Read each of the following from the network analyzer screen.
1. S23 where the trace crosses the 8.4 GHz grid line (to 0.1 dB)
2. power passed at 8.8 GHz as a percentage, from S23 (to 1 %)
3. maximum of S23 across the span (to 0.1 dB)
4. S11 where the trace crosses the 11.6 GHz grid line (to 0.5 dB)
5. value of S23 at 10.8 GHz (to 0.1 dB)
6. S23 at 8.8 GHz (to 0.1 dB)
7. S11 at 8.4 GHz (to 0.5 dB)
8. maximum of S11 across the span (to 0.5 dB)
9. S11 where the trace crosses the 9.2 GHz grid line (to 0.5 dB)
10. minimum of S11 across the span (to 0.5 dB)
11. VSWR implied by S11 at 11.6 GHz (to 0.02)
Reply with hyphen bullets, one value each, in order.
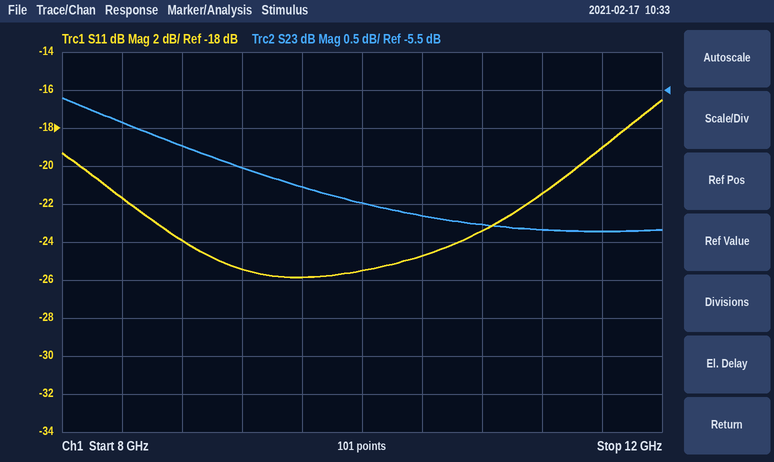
- -5.9 dB
- 24 %
- -5.6 dB
- -19.0 dB
- -7.3 dB
- -6.2 dB
- -21.5 dB
- -16.5 dB
- -25.5 dB
- -26.0 dB
- 1.26
